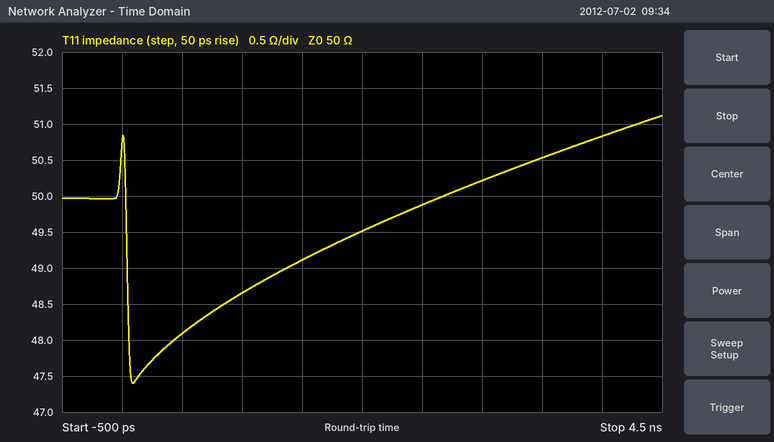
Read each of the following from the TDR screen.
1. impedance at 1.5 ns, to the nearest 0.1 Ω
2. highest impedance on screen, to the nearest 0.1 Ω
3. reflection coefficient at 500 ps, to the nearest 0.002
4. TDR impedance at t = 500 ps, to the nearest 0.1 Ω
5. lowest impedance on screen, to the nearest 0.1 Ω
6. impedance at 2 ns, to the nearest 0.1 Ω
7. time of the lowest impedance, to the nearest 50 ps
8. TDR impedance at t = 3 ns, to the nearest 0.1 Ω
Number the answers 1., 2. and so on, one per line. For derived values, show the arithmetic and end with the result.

1. 49.1 Ω
2. 51.1 Ω
3. (48.1 − 50)/(48.1 + 50) ≈ -0.0194, so -0.020 to the nearest 0.002
4. 48.1 Ω
5. 47.4 Ω
6. 49.5 Ω
7. 100 ps
8. 50.2 Ω
